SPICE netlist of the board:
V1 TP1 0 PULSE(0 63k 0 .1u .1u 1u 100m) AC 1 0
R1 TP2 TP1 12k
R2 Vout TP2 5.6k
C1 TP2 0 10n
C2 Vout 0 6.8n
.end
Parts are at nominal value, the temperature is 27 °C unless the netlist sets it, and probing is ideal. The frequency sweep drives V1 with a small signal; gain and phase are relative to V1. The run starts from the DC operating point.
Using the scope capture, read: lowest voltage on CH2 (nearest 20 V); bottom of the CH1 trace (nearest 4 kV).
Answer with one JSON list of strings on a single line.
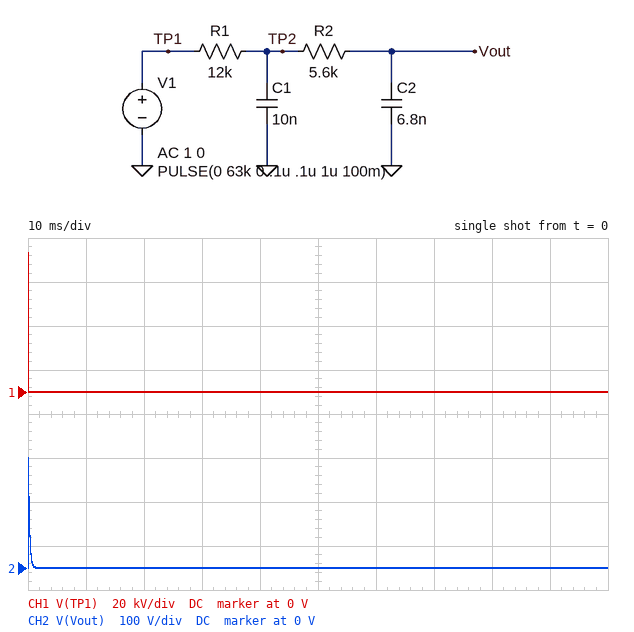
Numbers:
["0 V", "0 V"]
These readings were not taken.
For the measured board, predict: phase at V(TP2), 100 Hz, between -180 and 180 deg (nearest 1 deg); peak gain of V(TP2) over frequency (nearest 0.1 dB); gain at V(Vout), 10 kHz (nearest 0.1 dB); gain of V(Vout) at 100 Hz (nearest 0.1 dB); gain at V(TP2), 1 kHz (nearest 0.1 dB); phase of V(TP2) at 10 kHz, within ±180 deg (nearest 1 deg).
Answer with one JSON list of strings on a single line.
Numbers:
["-7 deg", "0 dB", "-27.1 dB", "-0.1 dB", "-4.4 dB", "-71 deg"]
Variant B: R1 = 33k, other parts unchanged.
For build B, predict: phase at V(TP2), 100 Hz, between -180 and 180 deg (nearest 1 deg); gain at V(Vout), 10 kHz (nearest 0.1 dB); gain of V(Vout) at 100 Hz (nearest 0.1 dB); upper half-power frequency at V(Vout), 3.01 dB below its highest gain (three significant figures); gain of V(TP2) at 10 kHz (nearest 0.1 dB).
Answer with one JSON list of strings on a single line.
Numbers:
["-19 deg", "-35.7 dB", "-0.5 dB", "279 Hz", "-27.5 dB"]
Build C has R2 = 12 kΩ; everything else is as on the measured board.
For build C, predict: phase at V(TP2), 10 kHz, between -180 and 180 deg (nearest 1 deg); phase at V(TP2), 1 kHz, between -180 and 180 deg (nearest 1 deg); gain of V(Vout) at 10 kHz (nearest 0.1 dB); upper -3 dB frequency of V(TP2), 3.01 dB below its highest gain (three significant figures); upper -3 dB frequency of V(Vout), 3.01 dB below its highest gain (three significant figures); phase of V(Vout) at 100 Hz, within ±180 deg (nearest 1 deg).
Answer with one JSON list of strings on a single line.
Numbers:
["-76 deg", "-44 deg", "-32.4 dB", "717 Hz", "638 Hz", "-10 deg"]
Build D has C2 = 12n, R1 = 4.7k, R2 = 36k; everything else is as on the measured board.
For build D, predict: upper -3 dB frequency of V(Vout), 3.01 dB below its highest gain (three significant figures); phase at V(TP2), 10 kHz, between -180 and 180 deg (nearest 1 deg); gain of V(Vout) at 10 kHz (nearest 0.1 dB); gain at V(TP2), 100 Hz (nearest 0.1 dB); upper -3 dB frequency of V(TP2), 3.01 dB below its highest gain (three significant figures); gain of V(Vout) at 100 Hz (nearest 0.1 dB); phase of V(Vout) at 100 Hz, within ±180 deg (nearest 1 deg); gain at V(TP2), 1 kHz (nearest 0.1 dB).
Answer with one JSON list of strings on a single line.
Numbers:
["320 Hz", "-69 deg", "-38.7 dB", "-0.1 dB", "2.83 kHz", "-0.4 dB", "-19 deg", "-1.3 dB"]
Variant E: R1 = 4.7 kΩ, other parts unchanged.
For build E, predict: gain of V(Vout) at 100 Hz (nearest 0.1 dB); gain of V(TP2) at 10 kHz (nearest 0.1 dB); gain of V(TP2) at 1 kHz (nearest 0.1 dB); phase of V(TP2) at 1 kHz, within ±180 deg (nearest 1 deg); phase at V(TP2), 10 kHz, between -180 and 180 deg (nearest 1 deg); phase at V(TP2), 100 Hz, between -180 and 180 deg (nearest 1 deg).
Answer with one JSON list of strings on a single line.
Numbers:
["0 dB", "-11.3 dB", "-1.2 dB", "-25 deg", "-62 deg", "-3 deg"]
